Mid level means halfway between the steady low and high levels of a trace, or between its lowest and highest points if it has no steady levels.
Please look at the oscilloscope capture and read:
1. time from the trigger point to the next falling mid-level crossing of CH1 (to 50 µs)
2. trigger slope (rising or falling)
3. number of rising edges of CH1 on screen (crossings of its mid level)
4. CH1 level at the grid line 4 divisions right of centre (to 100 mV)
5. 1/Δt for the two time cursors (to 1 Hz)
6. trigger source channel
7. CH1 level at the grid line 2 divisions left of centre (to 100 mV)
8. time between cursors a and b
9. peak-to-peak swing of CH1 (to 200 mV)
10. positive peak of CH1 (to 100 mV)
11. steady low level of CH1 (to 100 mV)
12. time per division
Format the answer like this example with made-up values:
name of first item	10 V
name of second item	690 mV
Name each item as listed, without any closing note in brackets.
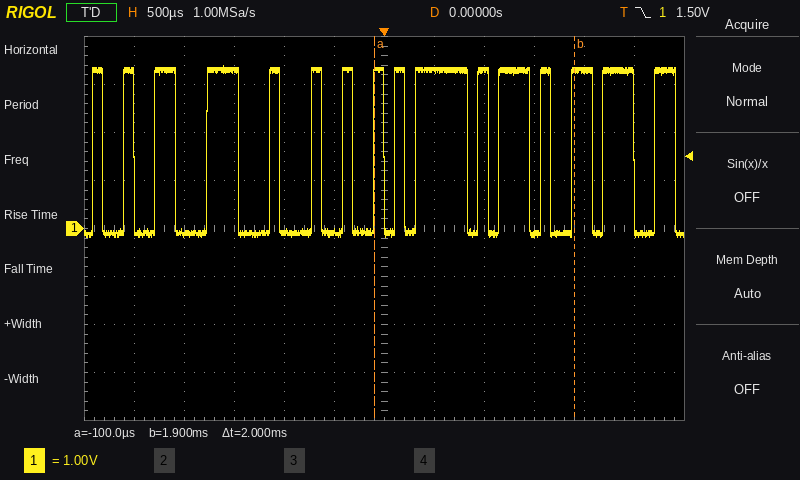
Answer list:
time from the trigger point to the next falling mid-level crossing of CH1	200 µs
trigger slope	falling
number of rising edges of CH1 on screen	16
CH1 level at the grid line 4 divisions right of centre	3.3 V
1/Δt for the two time cursors	500 Hz
trigger source channel	CH1
CH1 level at the grid line 2 divisions left of centre	-100 mV
time between cursors a and b	2 ms
peak-to-peak swing of CH1	3.6 V
positive peak of CH1	3.4 V
steady low level of CH1	-100 mV
time per division	500 µs
